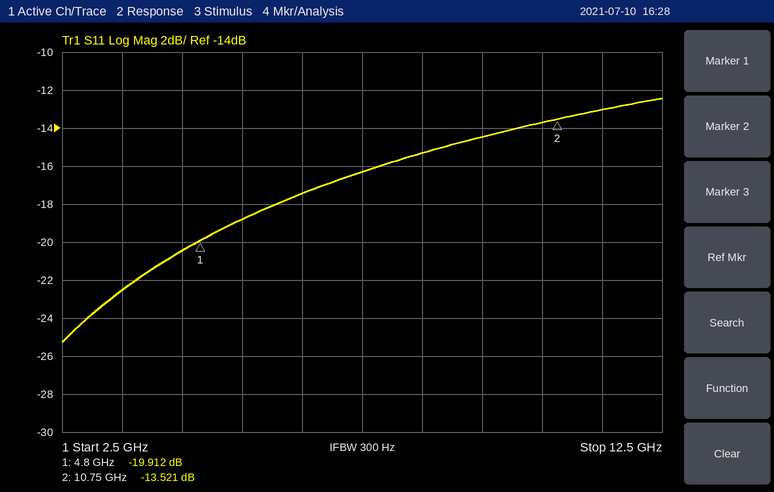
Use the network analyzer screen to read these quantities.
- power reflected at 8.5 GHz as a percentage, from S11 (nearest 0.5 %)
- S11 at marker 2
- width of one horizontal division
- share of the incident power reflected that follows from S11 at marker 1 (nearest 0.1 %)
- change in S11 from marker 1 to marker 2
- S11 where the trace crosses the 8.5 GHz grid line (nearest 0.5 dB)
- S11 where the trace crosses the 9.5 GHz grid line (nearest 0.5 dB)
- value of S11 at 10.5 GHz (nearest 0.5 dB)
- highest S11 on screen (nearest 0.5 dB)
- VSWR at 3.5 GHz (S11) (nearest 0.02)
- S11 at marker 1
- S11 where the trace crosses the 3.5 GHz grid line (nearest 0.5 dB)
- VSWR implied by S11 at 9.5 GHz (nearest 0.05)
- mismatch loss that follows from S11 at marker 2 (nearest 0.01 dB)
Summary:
3.0 %
-13.521 dB
1 GHz
1.0 %
6.391 dB
-15.5 dB
-14.5 dB
-13.5 dB
-12.5 dB
1.16
-19.912 dB
-22.5 dB
1.45
0.20 dB
